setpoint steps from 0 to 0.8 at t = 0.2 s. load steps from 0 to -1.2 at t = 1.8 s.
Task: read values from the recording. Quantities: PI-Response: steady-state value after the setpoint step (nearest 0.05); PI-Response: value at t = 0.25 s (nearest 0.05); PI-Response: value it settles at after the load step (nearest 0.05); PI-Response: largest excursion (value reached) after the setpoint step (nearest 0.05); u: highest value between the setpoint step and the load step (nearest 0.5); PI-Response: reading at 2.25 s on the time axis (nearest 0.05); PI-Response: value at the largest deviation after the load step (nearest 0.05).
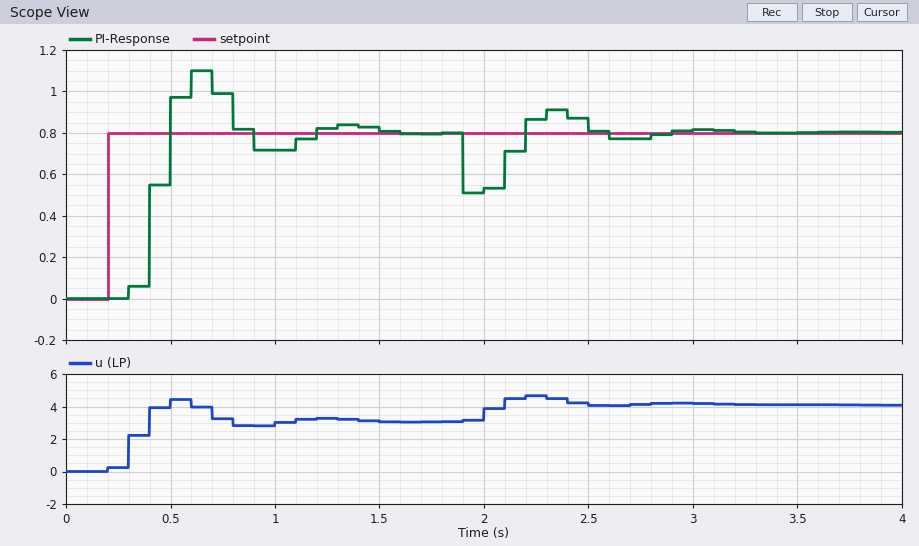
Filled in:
0.80
0.00
0.80
1.10
4.5
0.85
0.50
